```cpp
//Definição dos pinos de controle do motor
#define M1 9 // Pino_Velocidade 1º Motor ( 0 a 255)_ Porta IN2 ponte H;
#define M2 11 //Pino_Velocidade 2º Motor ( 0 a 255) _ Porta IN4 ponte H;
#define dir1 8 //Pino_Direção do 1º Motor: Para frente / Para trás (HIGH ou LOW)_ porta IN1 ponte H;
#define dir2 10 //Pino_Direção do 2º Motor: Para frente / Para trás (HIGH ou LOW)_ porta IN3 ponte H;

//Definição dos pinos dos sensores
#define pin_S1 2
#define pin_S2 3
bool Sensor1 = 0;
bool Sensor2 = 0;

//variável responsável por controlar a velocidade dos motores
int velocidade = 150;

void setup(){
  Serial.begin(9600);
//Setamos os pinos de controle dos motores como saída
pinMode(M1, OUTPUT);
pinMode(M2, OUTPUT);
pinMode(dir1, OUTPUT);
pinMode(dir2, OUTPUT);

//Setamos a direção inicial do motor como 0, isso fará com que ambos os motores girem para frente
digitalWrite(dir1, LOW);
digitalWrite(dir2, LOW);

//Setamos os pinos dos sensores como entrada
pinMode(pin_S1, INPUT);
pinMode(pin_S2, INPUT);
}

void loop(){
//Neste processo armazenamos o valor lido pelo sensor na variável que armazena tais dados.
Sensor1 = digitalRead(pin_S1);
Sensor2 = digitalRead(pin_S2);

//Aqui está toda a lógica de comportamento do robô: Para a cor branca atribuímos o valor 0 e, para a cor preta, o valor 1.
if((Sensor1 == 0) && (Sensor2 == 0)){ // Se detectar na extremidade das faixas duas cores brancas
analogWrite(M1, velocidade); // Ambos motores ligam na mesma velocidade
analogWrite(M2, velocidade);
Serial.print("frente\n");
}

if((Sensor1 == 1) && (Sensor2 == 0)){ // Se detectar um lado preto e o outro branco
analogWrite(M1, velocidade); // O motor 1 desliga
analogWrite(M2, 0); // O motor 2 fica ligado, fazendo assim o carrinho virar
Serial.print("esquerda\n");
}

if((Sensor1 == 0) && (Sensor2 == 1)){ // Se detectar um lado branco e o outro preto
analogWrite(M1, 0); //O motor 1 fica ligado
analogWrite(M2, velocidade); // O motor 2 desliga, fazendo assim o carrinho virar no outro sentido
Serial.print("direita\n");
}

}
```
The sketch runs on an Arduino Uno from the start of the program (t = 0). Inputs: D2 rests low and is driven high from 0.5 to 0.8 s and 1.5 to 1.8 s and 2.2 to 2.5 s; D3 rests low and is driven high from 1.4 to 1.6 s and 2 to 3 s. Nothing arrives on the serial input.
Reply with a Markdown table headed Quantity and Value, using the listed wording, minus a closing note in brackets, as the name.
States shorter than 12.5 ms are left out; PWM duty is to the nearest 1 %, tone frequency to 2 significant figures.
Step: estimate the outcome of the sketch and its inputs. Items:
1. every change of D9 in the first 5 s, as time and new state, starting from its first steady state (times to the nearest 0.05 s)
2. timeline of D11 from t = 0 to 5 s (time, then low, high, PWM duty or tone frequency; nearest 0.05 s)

| Quantity | Value |
|---|---|
| every change of D9 in the first 5 s, as time and new state, starting from its first steady state | 0 s PWM 59 %; 1.4 s low; 1.6 s PWM 59 %; 2 s low; 3 s PWM 59 % |
| timeline of D11 from t = 0 to 5 s | 0 s PWM 59 %; 0.5 s low; 0.8 s PWM 59 %; 1.6 s low; 1.8 s PWM 59 % |
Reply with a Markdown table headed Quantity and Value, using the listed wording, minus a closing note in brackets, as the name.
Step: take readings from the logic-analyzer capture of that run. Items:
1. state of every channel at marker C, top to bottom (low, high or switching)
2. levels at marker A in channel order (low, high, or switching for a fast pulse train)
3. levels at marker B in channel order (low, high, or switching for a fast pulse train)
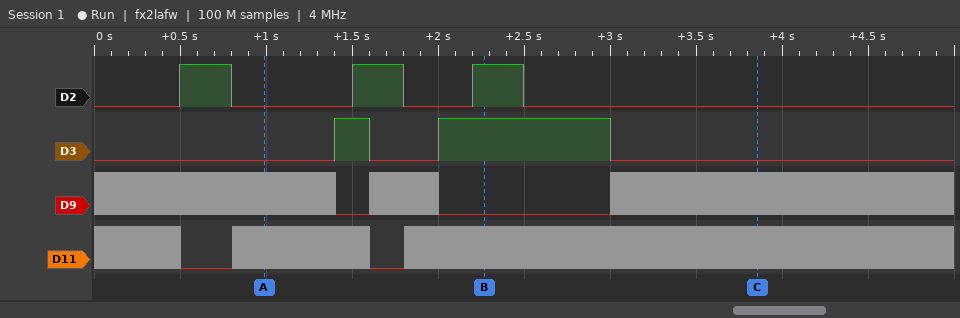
| Quantity | Value |
|---|---|
| state of every channel at marker C, top to bottom | D2 low, D3 low, D9 switching, D11 switching |
| levels at marker A in channel order | D2 low, D3 low, D9 switching, D11 switching |
| levels at marker B in channel order | D2 high, D3 high, D9 low, D11 switching |
